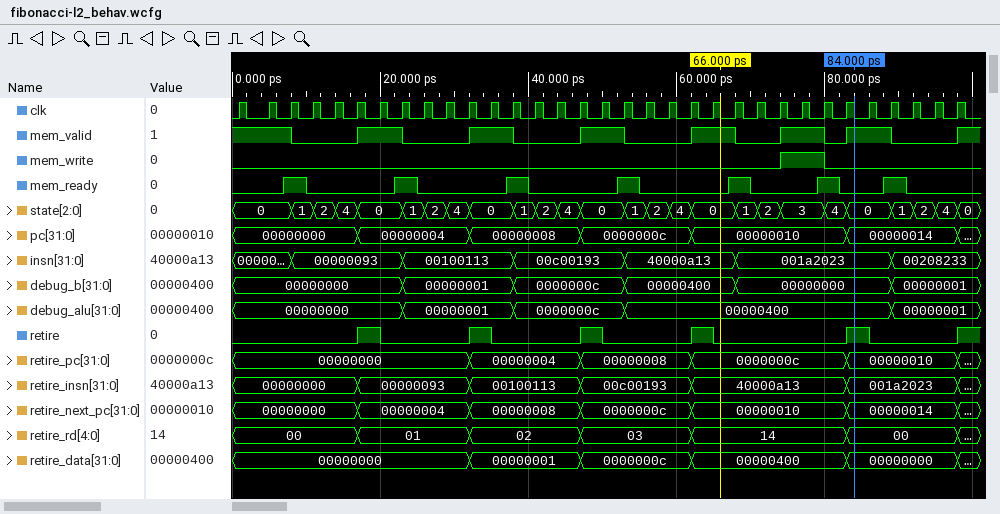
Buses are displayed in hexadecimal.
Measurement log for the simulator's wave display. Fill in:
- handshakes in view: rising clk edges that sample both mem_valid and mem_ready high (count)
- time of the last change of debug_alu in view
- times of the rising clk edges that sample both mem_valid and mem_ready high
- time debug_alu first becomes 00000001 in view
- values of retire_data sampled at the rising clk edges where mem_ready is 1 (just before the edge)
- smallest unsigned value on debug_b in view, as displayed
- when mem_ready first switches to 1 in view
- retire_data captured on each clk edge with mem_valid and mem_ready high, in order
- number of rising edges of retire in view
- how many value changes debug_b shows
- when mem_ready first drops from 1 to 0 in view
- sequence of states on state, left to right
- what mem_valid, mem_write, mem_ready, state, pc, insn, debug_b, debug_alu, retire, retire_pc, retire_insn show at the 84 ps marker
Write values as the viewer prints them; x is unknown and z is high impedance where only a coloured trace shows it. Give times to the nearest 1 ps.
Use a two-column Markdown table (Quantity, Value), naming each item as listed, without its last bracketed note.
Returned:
| Quantity | Value |
|---|---|
| handshakes in view: rising clk edges that sample both mem_valid and mem_ready high | 7 |
| time of the last change of debug_alu in view | 89 ps |
| times of the rising clk edges that sample both mem_valid and mem_ready high | 8 ps, 23 ps, 38 ps, 53 ps, 68 ps, 80 ps, 89 ps |
| time debug_alu first becomes 00000001 in view | 23 ps |
| values of retire_data sampled at the rising clk edges where mem_ready is 1 | 00000000, 00000000, 00000001, 0000000c, 00000400, 00000400, 00000000 |
| smallest unsigned value on debug_b in view, as displayed | 00000000 |
| when mem_ready first switches to 1 in view | 7 ps |
| retire_data captured on each clk edge with mem_valid and mem_ready high, in order | 00000000, 00000000, 00000001, 0000000c, 00000400, 00000400, 00000000 |
| number of rising edges of retire in view | 6 |
| how many value changes debug_b shows | 5 |
| when mem_ready first drops from 1 to 0 in view | 10 ps |
| sequence of states on state, left to right | 0, 1, 2, 4, 0, 1, 2, 4, 0, 1, 2, 4, 0, 1, 2, 4, 0, 1, 2, 3, 4, 0, 1, 2, 4, 0 |
| what mem_valid, mem_write, mem_ready, state, pc, insn, debug_b, debug_alu, retire, retire_pc, retire_insn show at the 84 ps marker | mem_valid=1, mem_write=0, mem_ready=0, state=0, pc=00000014, insn=001a2023, debug_b=00000000, debug_alu=00000400, retire=1, retire_pc=00000010, retire_insn=001a2023 |
